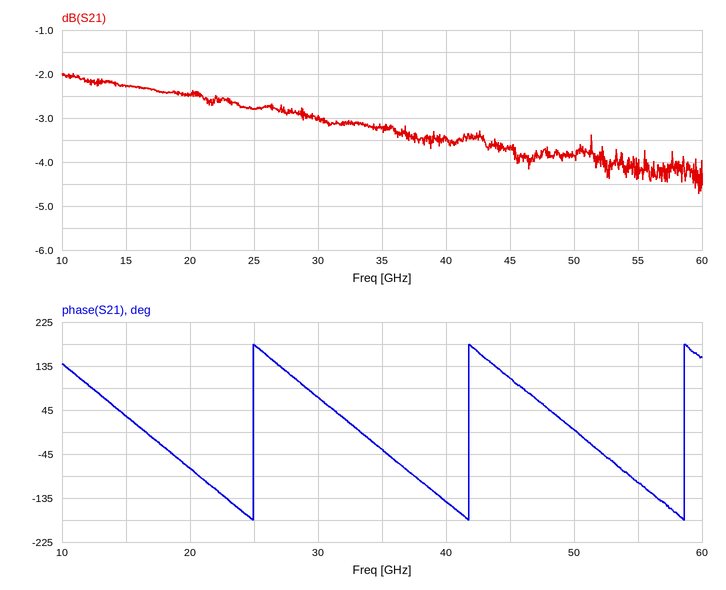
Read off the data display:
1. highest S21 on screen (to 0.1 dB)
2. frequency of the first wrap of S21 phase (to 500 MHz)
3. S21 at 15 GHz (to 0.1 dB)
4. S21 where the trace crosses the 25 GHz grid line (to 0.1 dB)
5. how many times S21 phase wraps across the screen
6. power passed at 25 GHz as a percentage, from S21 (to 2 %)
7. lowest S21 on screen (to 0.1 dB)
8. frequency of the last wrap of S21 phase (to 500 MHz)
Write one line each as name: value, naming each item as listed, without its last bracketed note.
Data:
highest S21 on screen: -2.0 dB
frequency of the first wrap of S21 phase: 25.0 GHz
S21 at 15 GHz: -2.3 dB
S21 where the trace crosses the 25 GHz grid line: -2.8 dB
how many times S21 phase wraps across the screen: 3
power passed at 25 GHz as a percentage, from S21: 52 %
lowest S21 on screen: -4.7 dB
frequency of the last wrap of S21 phase: 58.5 GHz
